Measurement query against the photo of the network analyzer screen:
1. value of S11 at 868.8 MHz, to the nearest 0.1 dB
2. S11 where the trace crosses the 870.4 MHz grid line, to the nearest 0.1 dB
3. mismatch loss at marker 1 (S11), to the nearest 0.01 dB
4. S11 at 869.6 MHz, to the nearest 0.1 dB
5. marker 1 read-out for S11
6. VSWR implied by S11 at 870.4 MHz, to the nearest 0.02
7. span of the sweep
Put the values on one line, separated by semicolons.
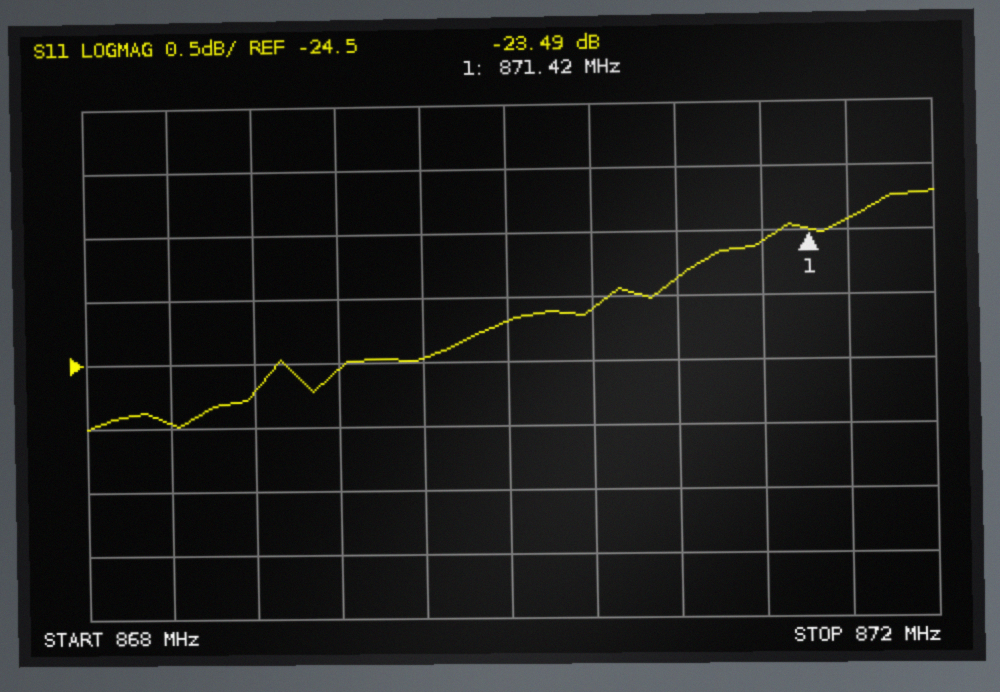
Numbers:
-24.7 dB; -24.1 dB; 0.02 dB; -24.5 dB; -23.49 dB; 1.14; 4 MHz
